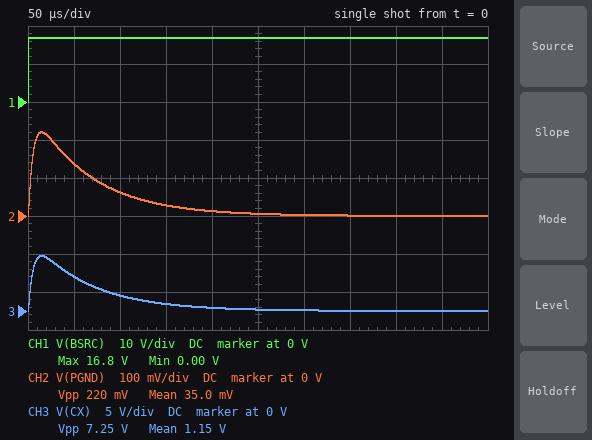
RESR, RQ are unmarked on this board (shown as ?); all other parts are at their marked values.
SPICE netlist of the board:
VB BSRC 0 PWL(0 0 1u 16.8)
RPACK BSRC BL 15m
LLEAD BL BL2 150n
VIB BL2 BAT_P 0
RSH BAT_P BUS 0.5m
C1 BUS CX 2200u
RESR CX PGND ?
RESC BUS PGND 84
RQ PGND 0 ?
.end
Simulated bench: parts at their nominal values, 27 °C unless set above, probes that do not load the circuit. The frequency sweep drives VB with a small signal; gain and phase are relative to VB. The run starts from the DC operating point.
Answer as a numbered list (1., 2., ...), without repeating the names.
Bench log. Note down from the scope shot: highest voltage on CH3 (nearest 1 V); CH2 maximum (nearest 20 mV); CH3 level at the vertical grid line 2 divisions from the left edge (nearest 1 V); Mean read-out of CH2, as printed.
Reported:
1. 7 V
2. 220 mV
3. 2 V
4. 35.0 mV
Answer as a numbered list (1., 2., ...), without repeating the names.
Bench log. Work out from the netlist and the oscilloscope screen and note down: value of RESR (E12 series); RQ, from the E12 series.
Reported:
1. 0.015 Ω
2. 470 µΩ
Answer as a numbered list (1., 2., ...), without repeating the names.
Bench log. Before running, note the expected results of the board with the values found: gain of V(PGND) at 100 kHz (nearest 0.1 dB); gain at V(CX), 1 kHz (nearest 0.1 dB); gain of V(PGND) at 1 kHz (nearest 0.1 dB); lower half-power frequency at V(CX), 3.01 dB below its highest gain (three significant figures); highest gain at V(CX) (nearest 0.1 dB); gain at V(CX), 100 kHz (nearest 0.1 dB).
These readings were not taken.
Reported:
1. -46.4 dB
2. -14.0 dB
3. -44.4 dB
4. 2.19 kHz
5. -6.0 dB
6. -16.1 dB
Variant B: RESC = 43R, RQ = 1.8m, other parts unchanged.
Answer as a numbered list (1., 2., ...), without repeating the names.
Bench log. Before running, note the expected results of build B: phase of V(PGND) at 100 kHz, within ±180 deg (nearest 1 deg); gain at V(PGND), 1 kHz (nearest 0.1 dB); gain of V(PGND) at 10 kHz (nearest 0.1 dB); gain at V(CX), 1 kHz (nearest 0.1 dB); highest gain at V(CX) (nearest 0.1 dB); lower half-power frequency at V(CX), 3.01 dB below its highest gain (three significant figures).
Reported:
1. -71 deg
2. -32.8 dB
3. -25.1 dB
4. -13.4 dB
5. -5.7 dB
6. 2.11 kHz
